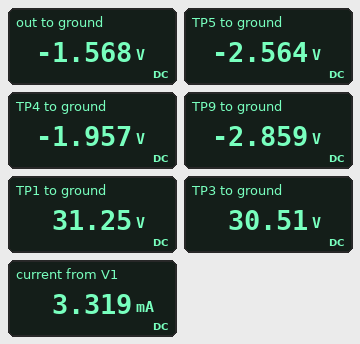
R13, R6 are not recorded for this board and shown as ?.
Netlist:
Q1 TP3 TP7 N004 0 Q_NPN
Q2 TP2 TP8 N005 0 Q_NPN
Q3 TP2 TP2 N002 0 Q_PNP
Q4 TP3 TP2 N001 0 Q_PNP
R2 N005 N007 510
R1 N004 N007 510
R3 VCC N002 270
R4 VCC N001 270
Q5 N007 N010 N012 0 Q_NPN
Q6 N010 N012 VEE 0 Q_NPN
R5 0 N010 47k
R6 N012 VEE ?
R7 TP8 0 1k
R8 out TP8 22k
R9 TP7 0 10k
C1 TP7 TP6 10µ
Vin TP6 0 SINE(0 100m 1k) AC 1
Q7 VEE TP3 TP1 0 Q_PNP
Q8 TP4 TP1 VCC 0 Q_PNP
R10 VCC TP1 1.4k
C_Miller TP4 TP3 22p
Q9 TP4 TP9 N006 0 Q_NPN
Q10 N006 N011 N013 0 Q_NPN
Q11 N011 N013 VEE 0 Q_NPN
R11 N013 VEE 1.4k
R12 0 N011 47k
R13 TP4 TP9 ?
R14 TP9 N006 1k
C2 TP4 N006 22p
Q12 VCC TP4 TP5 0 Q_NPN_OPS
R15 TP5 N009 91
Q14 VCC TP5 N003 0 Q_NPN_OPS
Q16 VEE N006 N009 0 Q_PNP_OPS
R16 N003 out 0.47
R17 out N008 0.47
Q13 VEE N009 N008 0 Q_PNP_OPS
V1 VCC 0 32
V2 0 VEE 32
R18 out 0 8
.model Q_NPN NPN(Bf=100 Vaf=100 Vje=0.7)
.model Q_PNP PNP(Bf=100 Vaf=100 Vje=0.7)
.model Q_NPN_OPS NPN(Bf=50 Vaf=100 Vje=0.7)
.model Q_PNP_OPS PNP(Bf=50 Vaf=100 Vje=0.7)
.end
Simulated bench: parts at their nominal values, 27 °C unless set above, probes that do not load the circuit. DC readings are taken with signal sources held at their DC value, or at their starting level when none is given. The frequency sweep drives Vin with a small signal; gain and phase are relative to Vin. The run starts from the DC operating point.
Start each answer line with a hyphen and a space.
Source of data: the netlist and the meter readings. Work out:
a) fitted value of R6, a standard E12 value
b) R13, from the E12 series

- 330 Ω
- 1.8 kΩ
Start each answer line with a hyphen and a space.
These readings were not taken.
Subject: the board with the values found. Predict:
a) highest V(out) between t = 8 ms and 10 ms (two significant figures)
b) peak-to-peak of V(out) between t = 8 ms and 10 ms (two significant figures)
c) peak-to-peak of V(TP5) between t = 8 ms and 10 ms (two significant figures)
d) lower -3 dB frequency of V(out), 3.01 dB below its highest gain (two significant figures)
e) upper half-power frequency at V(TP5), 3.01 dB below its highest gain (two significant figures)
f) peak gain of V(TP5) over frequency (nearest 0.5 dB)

- 730 mV
- 4.6 V
- 6.7 V
- 1.6 Hz
- 490 kHz
- 28.0 dB
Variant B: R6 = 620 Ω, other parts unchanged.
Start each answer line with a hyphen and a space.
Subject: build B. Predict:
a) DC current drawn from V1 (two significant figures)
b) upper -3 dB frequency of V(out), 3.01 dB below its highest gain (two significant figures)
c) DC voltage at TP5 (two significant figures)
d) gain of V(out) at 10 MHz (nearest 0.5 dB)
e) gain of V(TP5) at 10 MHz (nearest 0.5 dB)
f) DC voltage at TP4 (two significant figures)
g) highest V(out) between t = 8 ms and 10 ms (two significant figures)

- 2.3 mA
- 460 kHz
- -1.8 V
- 1.0 dB
- 2.0 dB
- -1.1 V
- 1.4 V
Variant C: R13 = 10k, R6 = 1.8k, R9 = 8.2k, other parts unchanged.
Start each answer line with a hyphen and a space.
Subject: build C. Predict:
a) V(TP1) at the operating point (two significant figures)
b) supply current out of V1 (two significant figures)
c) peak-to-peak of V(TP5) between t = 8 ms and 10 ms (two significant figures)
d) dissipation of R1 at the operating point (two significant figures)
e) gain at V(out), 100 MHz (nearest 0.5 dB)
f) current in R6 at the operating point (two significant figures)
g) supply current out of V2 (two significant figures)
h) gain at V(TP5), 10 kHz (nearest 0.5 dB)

- 31 V
- 18 mA
- 5.5 V
- 23 µW
- -18.5 dB
- 420 µA
- 53 mA
- 29.5 dB
